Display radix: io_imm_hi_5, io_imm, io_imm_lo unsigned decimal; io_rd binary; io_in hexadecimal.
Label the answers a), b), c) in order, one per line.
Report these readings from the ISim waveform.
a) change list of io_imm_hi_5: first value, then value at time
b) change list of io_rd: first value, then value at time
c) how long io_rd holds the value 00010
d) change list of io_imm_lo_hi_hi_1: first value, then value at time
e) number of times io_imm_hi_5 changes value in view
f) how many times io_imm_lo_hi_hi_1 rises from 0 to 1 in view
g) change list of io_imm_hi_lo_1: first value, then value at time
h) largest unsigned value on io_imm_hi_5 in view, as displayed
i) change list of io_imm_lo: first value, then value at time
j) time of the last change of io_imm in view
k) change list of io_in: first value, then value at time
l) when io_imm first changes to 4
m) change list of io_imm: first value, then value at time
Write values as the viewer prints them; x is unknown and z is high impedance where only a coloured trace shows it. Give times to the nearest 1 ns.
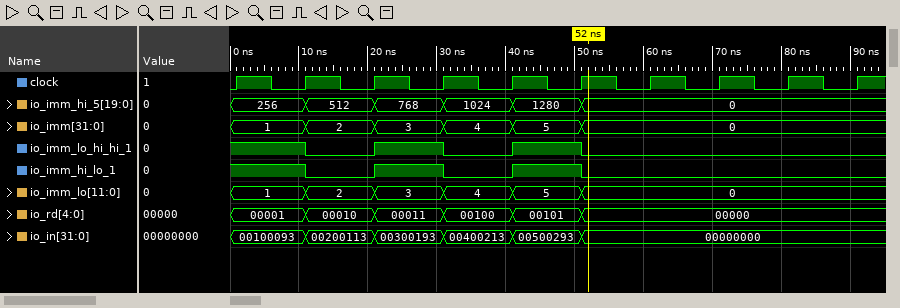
a) 256, 512 at 11 ns, 768 at 21 ns, 1024 at 31 ns, 1280 at 41 ns, 0 at 51 ns
b) 00001, 00010 at 11 ns, 00011 at 21 ns, 00100 at 31 ns, 00101 at 41 ns, 00000 at 51 ns
c) 10 ns
d) 1, 0 at 11 ns, 1 at 21 ns, 0 at 31 ns, 1 at 41 ns, 0 at 51 ns
e) 5
f) 2
g) 1, 0 at 11 ns, 1 at 21 ns, 0 at 31 ns, 1 at 41 ns, 0 at 51 ns
h) 1280
i) 1, 2 at 11 ns, 3 at 21 ns, 4 at 31 ns, 5 at 41 ns, 0 at 51 ns
j) 51 ns
k) 00100093, 00200113 at 11 ns, 00300193 at 21 ns, 00400213 at 31 ns, 00500293 at 41 ns, 00000000 at 51 ns
l) 31 ns
m) 1, 2 at 11 ns, 3 at 21 ns, 4 at 31 ns, 5 at 41 ns, 0 at 51 ns
